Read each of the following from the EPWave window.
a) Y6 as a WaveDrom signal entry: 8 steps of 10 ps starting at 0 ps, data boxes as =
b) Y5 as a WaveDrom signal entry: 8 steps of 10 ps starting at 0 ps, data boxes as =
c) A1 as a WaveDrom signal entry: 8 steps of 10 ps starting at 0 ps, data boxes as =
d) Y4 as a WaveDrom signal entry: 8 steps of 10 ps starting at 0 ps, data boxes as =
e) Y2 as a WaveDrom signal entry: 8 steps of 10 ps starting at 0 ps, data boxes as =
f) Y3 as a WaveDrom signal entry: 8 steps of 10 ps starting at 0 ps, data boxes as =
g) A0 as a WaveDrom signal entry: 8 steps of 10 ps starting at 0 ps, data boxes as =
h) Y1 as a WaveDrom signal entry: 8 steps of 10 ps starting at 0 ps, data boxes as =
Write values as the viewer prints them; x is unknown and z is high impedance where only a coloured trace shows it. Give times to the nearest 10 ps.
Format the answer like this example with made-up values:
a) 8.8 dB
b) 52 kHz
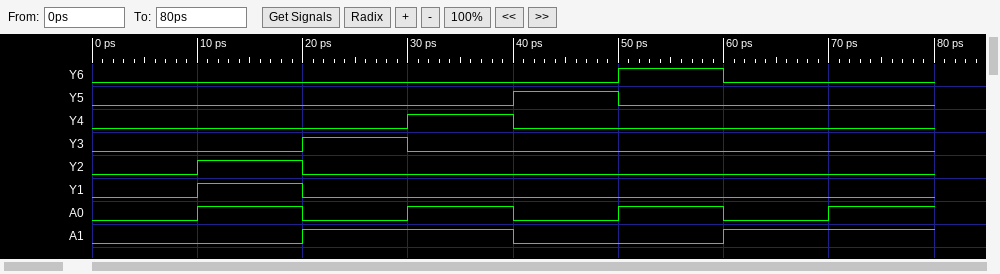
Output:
a) {name: 'Y6', wave: '0....10.'}
b) {name: 'Y5', wave: '0...10..'}
c) {name: 'A1', wave: '0.1.0.1.'}
d) {name: 'Y4', wave: '0..10...'}
e) {name: 'Y2', wave: '010.....'}
f) {name: 'Y3', wave: '0.10....'}
g) {name: 'A0', wave: '01010101'}
h) {name: 'Y1', wave: '010.....'}
